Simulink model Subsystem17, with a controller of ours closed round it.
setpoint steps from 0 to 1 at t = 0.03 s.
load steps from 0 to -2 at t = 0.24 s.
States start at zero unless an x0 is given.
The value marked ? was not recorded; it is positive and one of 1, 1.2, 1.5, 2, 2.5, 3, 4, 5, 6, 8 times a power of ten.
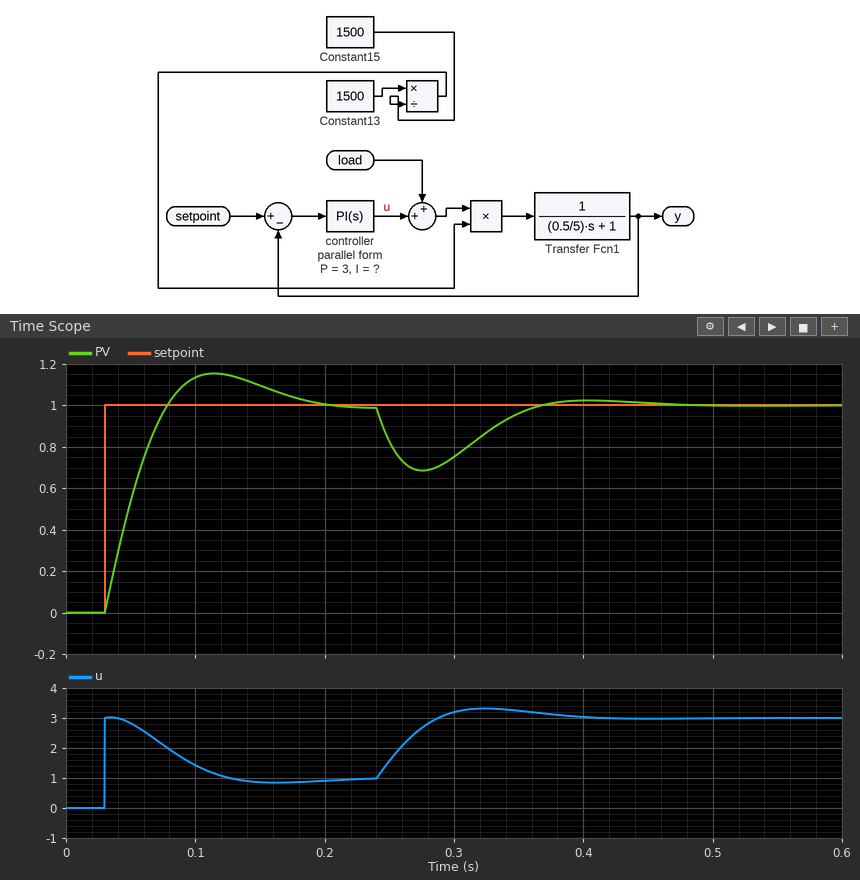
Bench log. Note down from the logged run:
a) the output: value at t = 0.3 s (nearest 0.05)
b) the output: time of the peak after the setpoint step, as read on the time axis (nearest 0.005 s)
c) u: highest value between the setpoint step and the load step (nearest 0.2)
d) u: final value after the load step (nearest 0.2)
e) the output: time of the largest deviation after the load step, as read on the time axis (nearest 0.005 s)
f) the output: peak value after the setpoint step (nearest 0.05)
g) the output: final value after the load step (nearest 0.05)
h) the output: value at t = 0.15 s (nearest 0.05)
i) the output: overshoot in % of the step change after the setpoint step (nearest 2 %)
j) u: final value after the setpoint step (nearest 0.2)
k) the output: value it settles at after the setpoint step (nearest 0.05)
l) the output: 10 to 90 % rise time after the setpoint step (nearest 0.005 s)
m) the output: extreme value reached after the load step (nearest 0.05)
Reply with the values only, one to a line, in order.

0.75
0.115 s
3.0
3.0
0.275 s
1.15
1.00
1.10
16 %
1.0
1.00
0.035 s
0.70
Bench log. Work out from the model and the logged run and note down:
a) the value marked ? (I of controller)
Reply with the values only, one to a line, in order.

100
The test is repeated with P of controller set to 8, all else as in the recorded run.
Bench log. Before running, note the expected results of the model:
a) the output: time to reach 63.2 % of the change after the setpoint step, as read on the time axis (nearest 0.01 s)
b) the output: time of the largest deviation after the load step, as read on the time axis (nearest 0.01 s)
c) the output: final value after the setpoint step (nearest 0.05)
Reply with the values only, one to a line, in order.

0.04 s
0.27 s
1.00
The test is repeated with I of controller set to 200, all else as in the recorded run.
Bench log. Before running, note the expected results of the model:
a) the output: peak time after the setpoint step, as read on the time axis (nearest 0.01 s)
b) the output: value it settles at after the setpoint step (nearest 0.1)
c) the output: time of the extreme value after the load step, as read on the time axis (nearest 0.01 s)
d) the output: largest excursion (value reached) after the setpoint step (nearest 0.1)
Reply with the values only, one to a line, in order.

0.09 s
1.0
0.27 s
1.3
